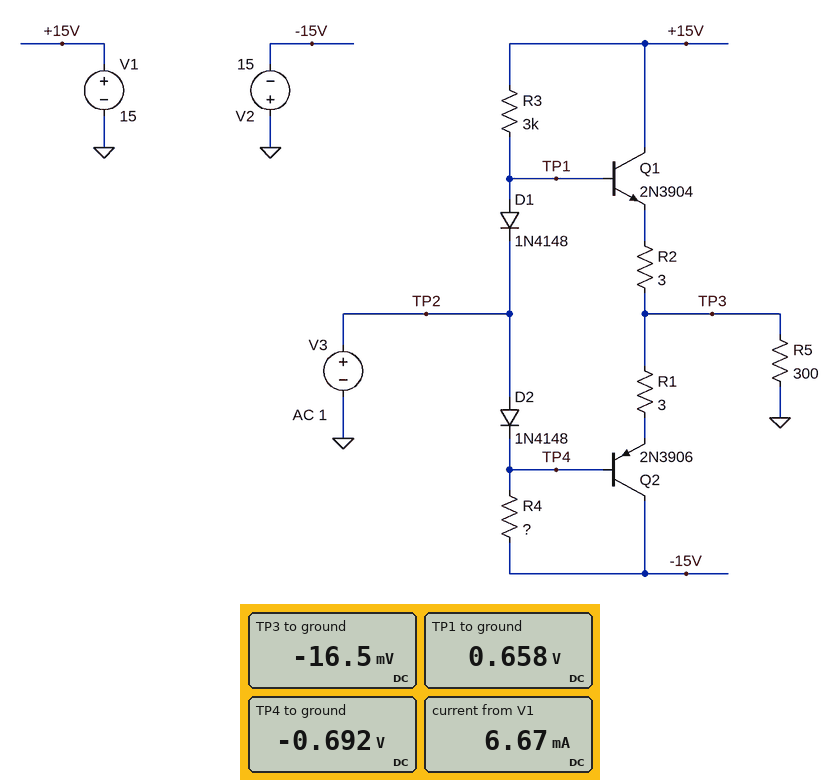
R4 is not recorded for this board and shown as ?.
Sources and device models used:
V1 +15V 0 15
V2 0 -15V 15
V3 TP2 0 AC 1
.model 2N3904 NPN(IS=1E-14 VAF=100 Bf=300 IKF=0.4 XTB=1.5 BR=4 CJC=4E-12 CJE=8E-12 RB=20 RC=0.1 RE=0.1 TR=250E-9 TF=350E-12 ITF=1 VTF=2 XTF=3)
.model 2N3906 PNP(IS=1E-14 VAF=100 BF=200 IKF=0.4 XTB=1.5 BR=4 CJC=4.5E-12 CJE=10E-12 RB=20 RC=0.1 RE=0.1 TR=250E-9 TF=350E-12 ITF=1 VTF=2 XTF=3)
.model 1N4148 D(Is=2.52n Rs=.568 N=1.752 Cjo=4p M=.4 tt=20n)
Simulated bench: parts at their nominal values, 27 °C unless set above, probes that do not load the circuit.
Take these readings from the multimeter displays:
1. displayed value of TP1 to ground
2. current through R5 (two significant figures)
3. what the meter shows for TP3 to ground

0.658 V
55 µA
-16.5 mV
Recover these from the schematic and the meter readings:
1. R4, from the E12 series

1.5 kΩ
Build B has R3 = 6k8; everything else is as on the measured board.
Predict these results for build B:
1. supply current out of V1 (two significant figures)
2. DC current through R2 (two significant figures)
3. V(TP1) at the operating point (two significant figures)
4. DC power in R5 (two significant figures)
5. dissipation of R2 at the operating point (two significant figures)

3.1 mA
970 µA
620 mV
4.0 µW
2.8 µW
